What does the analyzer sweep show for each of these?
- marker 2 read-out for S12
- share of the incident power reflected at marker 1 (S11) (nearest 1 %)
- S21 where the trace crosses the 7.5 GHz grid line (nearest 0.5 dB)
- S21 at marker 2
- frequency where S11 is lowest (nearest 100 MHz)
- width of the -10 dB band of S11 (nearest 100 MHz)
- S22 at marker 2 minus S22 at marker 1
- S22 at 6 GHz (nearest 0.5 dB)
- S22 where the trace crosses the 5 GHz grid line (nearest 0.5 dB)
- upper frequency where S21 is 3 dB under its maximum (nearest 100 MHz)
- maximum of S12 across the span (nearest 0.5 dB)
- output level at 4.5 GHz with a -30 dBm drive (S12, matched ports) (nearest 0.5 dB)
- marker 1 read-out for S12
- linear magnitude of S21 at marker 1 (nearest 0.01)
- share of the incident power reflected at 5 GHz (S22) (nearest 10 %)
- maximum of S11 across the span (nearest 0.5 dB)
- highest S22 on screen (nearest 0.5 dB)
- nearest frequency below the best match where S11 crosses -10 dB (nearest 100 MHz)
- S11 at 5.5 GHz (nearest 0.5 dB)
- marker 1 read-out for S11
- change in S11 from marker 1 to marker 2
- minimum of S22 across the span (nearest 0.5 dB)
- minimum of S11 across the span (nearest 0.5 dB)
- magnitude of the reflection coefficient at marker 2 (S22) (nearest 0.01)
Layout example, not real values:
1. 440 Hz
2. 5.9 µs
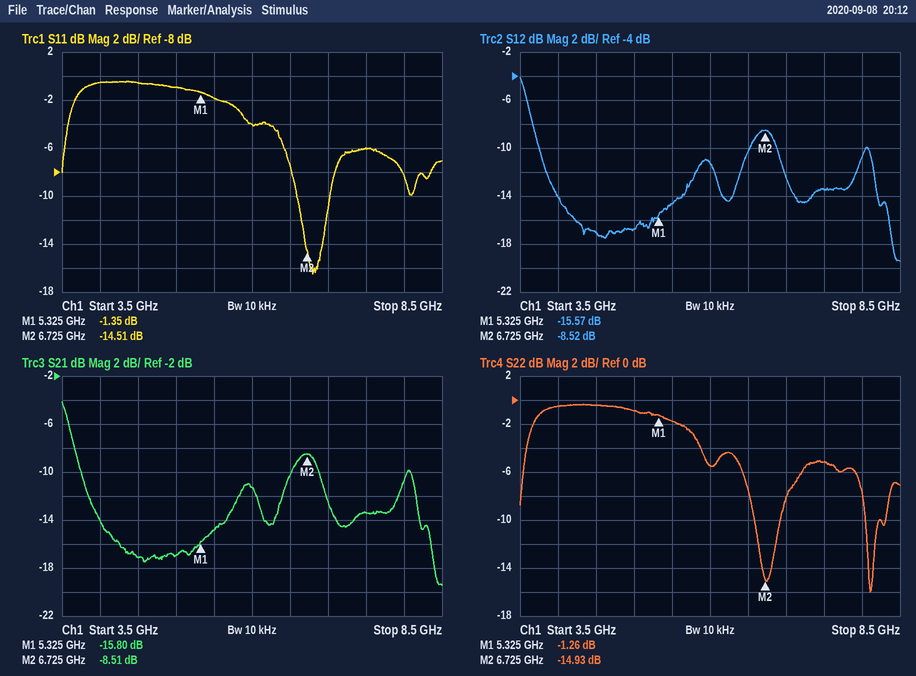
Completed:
1. -8.52 dB
2. 73 %
3. -13.5 dB
4. -8.51 dB
5. 6.8 GHz
6. 400 MHz
7. -13.67 dB
8. -5.5 dB
9. -1.0 dB
10. 3.6 GHz
11. -4.0 dB
12. -47.0 dBm
13. -15.57 dB
14. 0.16
15. 80 %
16. -0.5 dB
17. -0.5 dB
18. 6.6 GHz
19. -2.0 dB
20. -1.35 dB
21. -13.16 dB
22. -16.0 dB
23. -16.5 dB
24. 0.18
